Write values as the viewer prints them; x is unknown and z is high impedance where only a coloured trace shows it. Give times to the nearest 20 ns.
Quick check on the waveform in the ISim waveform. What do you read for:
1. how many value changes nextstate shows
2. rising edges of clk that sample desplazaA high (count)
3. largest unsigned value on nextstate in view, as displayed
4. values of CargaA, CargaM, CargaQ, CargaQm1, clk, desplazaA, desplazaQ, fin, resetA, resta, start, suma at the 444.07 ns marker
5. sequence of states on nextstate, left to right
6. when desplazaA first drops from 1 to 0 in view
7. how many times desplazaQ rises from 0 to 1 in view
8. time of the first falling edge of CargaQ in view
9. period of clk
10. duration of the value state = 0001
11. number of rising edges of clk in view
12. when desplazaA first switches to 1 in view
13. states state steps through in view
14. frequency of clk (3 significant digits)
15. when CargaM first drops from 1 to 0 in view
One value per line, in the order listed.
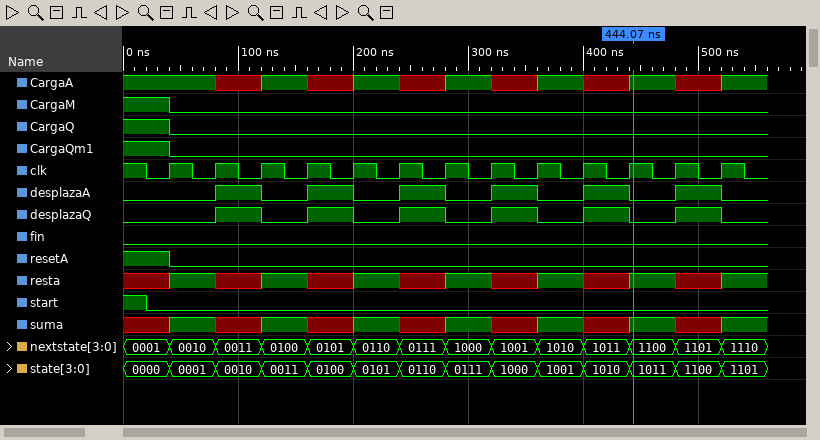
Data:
13
6
1110
CargaA=1, CargaM=0, CargaQ=0, CargaQm1=0, clk=1, desplazaA=0, desplazaQ=0, fin=0, resetA=0, resta=1, start=0, suma=1
0001, 0010, 0011, 0100, 0101, 0110, 0111, 1000, 1001, 1010, 1011, 1100, 1101, 1110
120 ns
6
40 ns
40 ns
40 ns
13
80 ns
0000, 0001, 0010, 0011, 0100, 0101, 0110, 0111, 1000, 1001, 1010, 1011, 1100, 1101
25.0 MHz
40 ns
